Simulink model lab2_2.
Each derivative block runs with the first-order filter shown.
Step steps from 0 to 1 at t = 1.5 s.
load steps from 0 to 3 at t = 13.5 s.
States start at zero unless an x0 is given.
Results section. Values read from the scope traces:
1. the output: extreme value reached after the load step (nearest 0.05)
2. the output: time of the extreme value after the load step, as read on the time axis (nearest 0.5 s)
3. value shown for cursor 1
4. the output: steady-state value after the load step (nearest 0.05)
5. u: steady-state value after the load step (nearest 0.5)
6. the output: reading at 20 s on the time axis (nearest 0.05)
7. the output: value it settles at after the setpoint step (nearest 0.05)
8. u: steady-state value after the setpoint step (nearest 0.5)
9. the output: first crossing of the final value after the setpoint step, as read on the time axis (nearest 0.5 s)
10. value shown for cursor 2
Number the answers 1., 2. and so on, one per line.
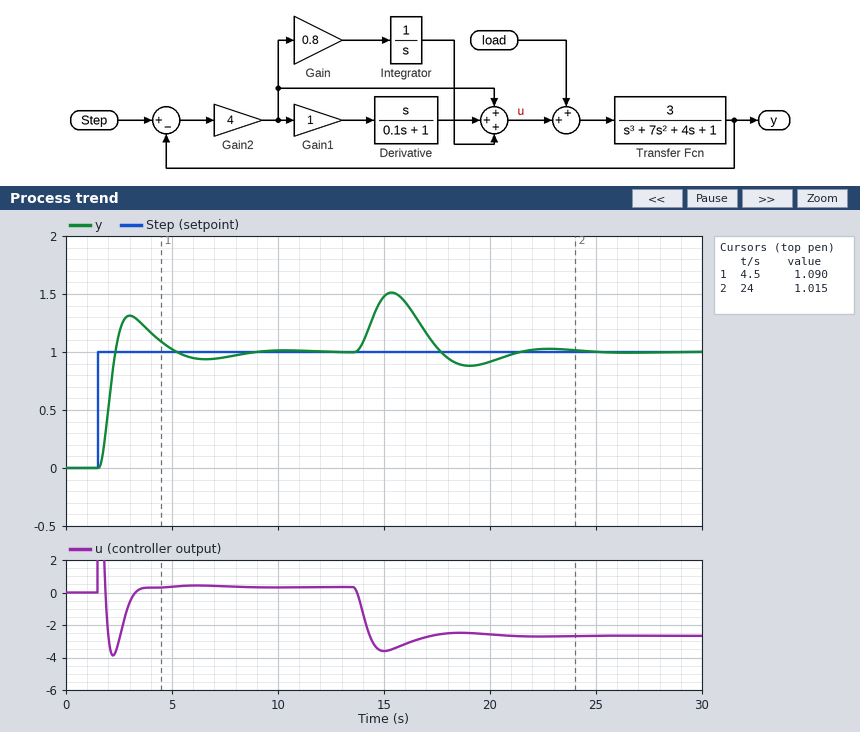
1. 1.50
2. 15.5 s
3. 1.090
4. 1.00
5. -2.5
6. 0.90
7. 1.00
8. 0.5
9. 2.5 s
10. 1.015
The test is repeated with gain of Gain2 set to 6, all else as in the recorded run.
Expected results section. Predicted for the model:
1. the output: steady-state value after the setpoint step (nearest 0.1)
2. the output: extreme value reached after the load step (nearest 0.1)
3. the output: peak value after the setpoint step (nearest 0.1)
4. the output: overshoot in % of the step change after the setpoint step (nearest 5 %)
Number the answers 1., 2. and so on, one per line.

1. 1.0
2. 1.3
3. 1.4
4. 35 %
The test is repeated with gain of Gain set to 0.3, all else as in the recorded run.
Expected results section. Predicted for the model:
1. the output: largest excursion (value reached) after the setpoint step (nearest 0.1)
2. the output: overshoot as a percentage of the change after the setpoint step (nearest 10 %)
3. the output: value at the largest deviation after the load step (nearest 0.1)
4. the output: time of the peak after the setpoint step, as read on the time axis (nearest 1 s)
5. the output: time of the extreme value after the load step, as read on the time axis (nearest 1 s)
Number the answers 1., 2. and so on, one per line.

1. 1.2
2. 20 %
3. 1.6
4. 3 s
5. 16 s
